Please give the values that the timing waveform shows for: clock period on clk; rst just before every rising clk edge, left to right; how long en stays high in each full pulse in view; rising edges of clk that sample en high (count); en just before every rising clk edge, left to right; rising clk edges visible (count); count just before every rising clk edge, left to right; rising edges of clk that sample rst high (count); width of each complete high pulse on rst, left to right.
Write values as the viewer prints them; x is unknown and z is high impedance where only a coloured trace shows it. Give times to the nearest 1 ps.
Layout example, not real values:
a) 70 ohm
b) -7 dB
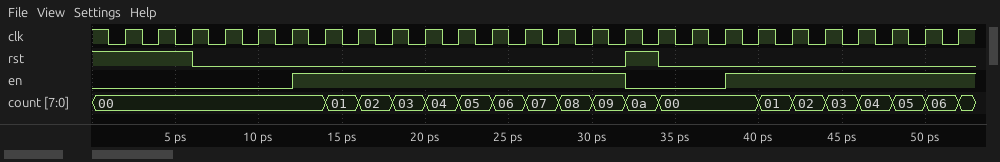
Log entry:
a) 2 ps
b) 1 1 1 0 0 0 0 0 0 0 0 0 0 0 0 0 1 0 0 0 0 0 0 0 0 0
c) 20 ps
d) 17
e) 0 0 0 0 0 0 1 1 1 1 1 1 1 1 1 1 0 0 0 1 1 1 1 1 1 1
f) 26
g) 00, 00, 00, 00, 00, 00, 00, 01, 02, 03, 04, 05, 06, 07, 08, 09, 0a, 00, 00, 00, 01, 02, 03, 04, 05, 06
h) 4
i) 2 ps
